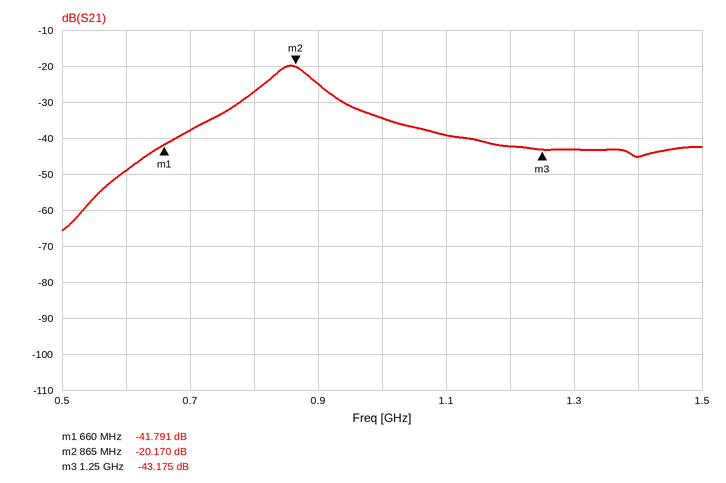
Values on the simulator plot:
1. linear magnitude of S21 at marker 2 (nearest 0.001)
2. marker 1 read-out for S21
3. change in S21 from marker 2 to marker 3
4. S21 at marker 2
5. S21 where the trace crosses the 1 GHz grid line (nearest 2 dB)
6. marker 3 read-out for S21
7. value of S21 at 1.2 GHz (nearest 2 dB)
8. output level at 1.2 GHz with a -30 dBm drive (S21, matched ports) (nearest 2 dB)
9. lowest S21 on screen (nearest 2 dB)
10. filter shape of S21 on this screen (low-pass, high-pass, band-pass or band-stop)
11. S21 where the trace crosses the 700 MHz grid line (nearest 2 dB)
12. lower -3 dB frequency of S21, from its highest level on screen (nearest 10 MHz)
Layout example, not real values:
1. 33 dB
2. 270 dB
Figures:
1. 0.098
2. -41.791 dB
3. -23.005 dB
4. -20.170 dB
5. -34 dB
6. -43.175 dB
7. -42 dB
8. -72 dBm
9. -66 dB
10. band-pass
11. -38 dB
12. 830 MHz
